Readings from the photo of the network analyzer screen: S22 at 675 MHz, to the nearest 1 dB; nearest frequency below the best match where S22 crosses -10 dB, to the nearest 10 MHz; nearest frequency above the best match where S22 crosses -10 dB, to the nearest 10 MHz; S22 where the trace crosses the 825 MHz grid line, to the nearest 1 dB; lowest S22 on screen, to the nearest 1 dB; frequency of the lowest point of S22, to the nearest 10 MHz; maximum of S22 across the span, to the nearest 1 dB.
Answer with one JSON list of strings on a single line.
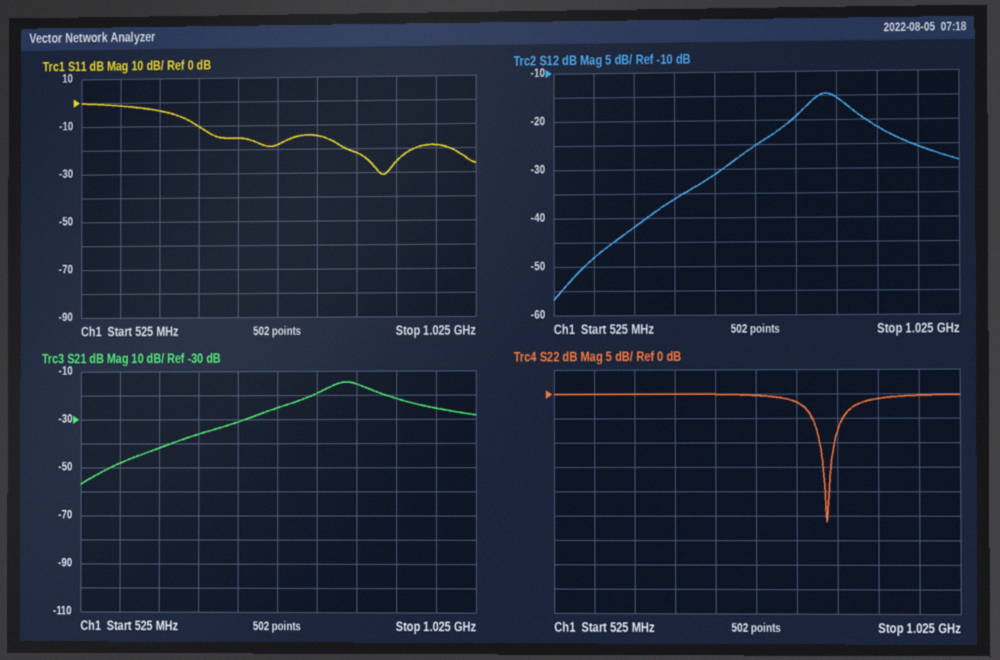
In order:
["0 dB", "850 MHz", "870 MHz", "-2 dB", "-26 dB", "860 MHz", "0 dB"]
